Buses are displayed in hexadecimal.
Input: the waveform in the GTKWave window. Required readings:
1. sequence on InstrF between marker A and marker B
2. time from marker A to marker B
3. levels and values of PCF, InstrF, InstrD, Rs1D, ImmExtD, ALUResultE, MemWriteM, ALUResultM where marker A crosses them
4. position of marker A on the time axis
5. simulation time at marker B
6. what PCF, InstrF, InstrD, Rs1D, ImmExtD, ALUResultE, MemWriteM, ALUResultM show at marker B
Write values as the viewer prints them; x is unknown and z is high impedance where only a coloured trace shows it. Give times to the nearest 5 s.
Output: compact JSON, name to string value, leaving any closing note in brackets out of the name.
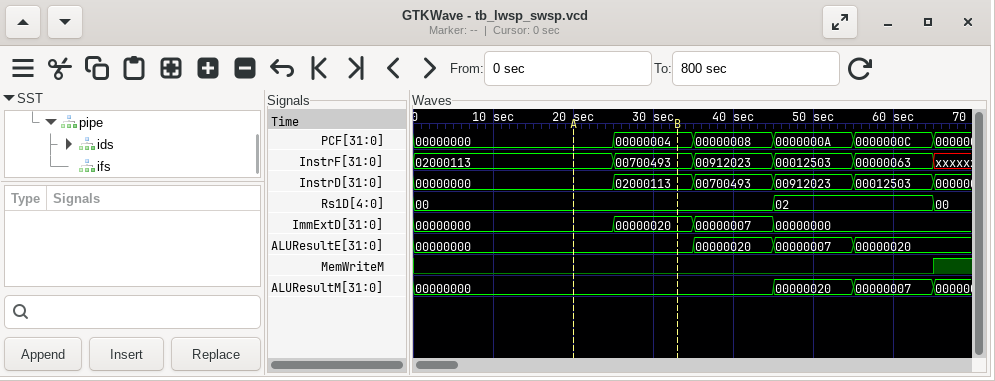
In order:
{"sequence on InstrF between marker A and marker B": "02000113, 00700493", "time from marker A to marker B": "15 s", "levels and values of PCF, InstrF, InstrD, Rs1D, ImmExtD, ALUResultE, MemWriteM, ALUResultM where marker A crosses them": "PCF=00000000, InstrF=02000113, InstrD=00000000, Rs1D=00, ImmExtD=00000000, ALUResultE=00000000, MemWriteM=0, ALUResultM=00000000", "position of marker A on the time axis": "20 s", "simulation time at marker B": "35 s", "what PCF, InstrF, InstrD, Rs1D, ImmExtD, ALUResultE, MemWriteM, ALUResultM show at marker B": "PCF=00000004, InstrF=00700493, InstrD=02000113, Rs1D=00, ImmExtD=00000020, ALUResultE=00000000, MemWriteM=0, ALUResultM=00000000"}
